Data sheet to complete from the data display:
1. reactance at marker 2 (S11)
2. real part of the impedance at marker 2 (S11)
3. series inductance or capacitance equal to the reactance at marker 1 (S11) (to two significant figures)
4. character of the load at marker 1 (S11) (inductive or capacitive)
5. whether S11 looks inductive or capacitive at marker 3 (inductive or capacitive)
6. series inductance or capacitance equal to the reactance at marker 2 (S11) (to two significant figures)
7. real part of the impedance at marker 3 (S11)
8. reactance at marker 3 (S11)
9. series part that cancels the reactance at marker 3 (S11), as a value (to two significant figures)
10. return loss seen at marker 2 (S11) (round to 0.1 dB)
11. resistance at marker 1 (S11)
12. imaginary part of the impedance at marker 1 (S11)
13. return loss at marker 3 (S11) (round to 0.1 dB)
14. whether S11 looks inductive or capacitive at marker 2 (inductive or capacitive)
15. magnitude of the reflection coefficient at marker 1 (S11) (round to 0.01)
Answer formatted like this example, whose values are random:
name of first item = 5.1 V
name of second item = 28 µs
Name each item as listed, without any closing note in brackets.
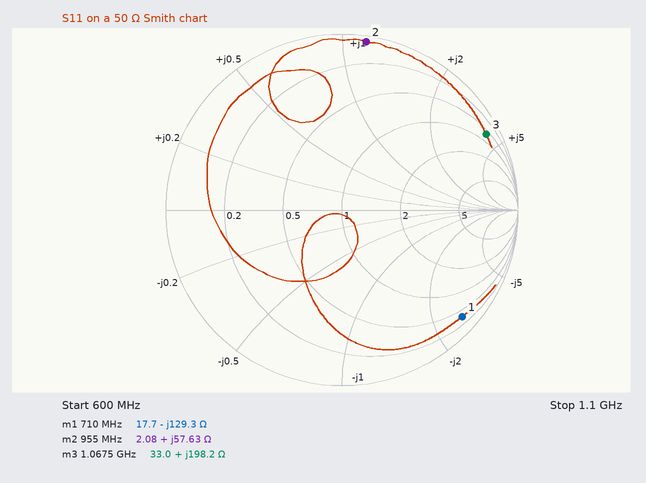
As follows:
reactance at marker 2 = +57.63 Ω
real part of the impedance at marker 2 = 2.08 Ω
series inductance or capacitance equal to the reactance at marker 1 (S11) = 1.7 pF
character of the load at marker 1 (S11) = capacitive
whether S11 looks inductive or capacitive at marker 3 = inductive
series inductance or capacitance equal to the reactance at marker 2 (S11) = 9.6 nH
real part of the impedance at marker 3 = 33.0 Ω
reactance at marker 3 = +198.2 Ω
series part that cancels the reactance at marker 3 (S11), as a value = 750 fF
return loss seen at marker 2 (S11) = 0.3 dB
resistance at marker 1 = 17.7 Ω
imaginary part of the impedance at marker 1 = -129.3 Ω
return loss at marker 3 (S11) = 0.7 dB
whether S11 looks inductive or capacitive at marker 2 = inductive
magnitude of the reflection coefficient at marker 1 (S11) = 0.91
